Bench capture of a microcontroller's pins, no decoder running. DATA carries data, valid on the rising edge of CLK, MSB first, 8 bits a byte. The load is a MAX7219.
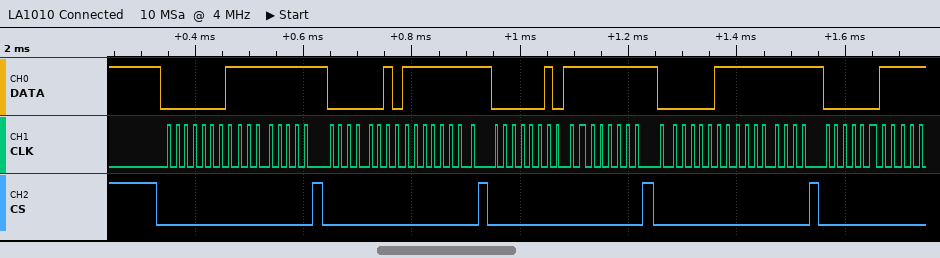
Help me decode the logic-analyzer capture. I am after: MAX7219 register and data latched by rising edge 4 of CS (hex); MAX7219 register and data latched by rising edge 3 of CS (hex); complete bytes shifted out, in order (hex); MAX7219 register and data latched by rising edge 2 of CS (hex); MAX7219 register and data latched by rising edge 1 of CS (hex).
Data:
register 0x3, data 0xFF
register 0x2, data 0xFF
01 FF 02 FF 02 FF 03 FF 03
register 0x2, data 0xFF
register 0x1, data 0xFF
